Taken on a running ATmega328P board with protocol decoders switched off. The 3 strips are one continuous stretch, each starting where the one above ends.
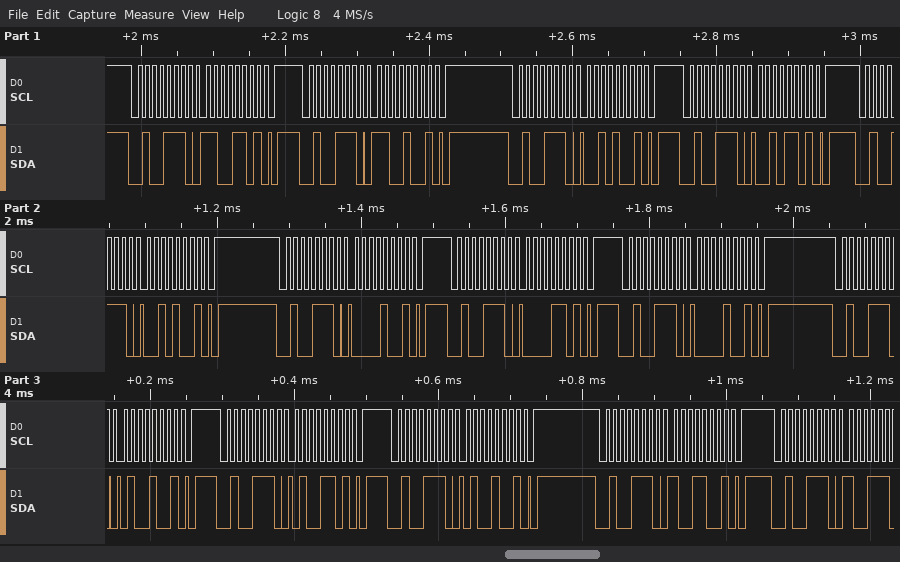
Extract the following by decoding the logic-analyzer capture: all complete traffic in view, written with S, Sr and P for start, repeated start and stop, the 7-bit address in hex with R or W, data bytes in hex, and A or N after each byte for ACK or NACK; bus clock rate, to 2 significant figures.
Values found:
S 27W A CD A P S 27W A C9 A P S 27W A 29 A P S 27W A 2D A P S 27W A 29 A P S 27W A 09 A P S 27W A 0D A P S 27W A 09 A P S 27W A 49 A P S 27W A 4D A P S 27W A 49 A P S 27W A 99 A P S 27W A
100 kHz
